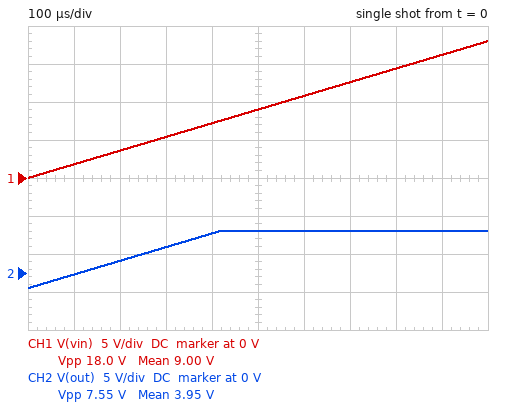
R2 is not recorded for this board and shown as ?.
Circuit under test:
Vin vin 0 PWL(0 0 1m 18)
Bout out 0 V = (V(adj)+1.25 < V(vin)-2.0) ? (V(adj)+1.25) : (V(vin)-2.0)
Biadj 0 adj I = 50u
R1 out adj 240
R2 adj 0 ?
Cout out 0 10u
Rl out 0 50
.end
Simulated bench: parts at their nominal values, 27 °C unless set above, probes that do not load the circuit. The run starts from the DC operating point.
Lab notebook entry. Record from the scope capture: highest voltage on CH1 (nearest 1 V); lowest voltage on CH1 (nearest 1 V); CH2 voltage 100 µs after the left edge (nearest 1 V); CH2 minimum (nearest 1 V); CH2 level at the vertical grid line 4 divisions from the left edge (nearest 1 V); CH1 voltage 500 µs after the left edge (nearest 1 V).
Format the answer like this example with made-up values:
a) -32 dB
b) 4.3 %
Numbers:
a) 18 V
b) 0 V
c) 0 V
d) -2 V
e) 5 V
f) 9 V
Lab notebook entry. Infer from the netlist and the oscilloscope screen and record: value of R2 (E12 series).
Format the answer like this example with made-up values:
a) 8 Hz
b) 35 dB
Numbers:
a) 820 Ω
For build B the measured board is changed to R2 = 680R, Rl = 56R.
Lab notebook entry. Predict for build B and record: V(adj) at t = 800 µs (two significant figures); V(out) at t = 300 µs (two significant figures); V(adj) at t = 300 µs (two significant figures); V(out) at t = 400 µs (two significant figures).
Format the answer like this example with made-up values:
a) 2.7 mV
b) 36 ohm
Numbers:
a) 3.6 V
b) 3.4 V
c) 2.5 V
d) 4.8 V
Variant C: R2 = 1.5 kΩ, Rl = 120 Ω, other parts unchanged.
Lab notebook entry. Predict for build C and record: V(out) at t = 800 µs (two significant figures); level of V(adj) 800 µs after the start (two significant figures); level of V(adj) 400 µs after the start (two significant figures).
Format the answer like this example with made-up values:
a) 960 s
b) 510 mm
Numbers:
a) 9.1 V
b) 7.9 V
c) 4.5 V
